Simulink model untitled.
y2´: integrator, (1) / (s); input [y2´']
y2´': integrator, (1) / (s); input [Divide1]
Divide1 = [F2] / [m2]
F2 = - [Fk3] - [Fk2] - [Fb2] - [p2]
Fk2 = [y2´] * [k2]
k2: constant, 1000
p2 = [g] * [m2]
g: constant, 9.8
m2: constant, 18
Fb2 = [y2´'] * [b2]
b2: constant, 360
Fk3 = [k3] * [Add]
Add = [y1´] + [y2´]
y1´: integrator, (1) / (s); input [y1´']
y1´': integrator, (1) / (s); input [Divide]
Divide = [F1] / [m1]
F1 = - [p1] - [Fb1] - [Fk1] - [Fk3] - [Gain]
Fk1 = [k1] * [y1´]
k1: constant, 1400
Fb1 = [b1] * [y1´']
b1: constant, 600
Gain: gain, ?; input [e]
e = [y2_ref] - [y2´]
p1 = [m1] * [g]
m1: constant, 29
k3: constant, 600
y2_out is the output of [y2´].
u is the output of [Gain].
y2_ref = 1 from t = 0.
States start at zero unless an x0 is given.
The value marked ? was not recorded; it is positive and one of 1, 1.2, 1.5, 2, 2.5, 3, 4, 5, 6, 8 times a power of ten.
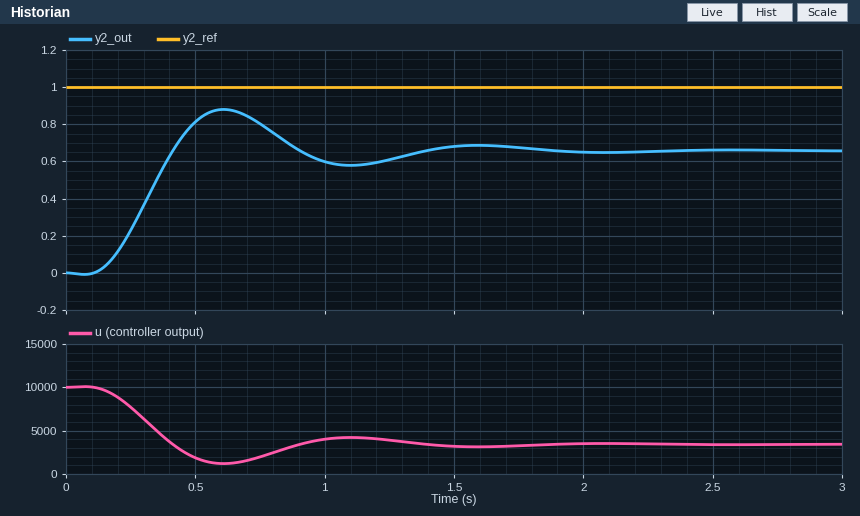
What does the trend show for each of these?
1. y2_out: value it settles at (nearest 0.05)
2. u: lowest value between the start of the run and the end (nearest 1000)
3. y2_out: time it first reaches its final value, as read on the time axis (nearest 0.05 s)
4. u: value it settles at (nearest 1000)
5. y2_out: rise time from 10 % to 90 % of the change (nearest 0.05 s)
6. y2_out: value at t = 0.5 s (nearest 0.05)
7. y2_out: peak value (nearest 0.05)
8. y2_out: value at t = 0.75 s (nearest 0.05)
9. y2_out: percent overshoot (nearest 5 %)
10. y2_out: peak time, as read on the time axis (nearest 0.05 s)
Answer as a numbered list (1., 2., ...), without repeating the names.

1. 0.65
2. 1000
3. 0.40 s
4. 3000
5. 0.20 s
6. 0.80
7. 0.90
8. 0.80
9. 35 %
10. 0.60 s
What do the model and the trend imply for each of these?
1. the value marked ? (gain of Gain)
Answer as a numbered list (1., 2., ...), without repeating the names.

1. 10000
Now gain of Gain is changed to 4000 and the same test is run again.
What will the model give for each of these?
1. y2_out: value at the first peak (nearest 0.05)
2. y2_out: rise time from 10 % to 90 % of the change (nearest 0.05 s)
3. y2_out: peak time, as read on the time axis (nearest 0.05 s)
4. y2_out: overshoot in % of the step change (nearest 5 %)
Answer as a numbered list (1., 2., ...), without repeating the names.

1. 0.45
2. 0.35 s
3. 0.85 s
4. 10 %
